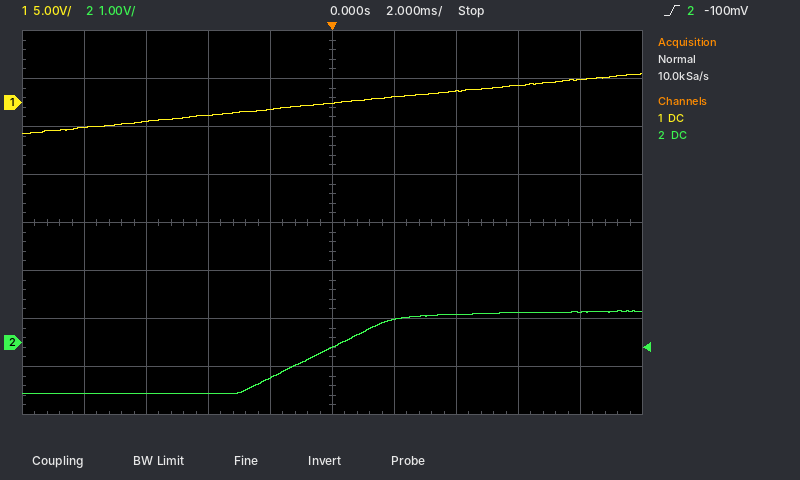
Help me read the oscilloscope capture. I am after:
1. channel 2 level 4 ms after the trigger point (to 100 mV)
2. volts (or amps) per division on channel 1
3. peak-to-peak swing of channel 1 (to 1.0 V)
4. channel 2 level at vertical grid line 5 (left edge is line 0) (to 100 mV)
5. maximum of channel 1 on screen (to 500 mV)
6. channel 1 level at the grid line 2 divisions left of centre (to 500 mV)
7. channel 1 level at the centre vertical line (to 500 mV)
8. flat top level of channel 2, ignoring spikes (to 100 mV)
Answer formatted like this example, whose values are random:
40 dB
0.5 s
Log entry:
600 mV
5 V
6.0 V
-100 mV
3.0 V
-1.5 V
0.0 V
600 mV
